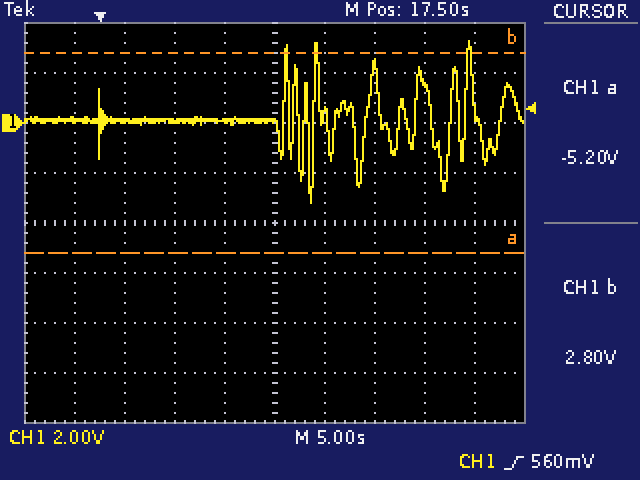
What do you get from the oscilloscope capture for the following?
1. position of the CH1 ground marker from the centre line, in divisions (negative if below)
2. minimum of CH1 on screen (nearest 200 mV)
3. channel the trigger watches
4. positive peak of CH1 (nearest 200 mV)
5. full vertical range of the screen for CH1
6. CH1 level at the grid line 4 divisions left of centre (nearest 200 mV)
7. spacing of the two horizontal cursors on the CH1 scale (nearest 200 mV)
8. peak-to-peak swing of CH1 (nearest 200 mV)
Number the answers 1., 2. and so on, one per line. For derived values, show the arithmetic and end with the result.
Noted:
1. +2.0 div
2. -3.2 V
3. CH1
4. 3.2 V
5. 16 V
6. 200 mV
7. 8.0 V
8. 3.2 V − (-3.2 V) = 6.4 V
